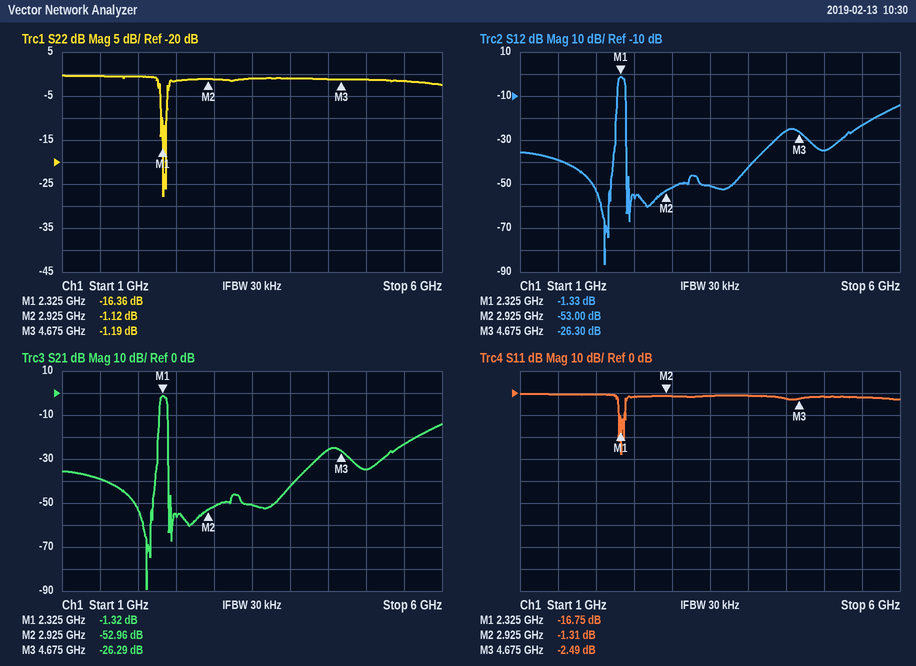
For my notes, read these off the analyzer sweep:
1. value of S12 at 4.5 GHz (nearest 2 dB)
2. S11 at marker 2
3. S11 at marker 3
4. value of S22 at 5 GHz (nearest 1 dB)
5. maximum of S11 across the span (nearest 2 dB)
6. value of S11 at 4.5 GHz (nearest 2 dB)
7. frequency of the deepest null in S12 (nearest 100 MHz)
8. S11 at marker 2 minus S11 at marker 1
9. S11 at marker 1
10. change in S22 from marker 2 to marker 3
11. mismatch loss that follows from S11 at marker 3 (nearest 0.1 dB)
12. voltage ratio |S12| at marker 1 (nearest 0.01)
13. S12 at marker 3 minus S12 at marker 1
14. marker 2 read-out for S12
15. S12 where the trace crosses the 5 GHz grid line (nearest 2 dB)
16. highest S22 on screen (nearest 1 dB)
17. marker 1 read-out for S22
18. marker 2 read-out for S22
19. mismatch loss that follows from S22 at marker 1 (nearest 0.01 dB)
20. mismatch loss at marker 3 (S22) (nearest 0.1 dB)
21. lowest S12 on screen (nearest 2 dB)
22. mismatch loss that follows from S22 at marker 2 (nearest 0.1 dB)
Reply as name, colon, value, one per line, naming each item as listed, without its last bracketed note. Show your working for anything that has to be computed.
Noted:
value of S12 at 4.5 GHz: -26 dB
S11 at marker 2: -1.31 dB
S11 at marker 3: -2.49 dB
value of S22 at 5 GHz: -1 dB
maximum of S11 across the span: 0 dB
value of S11 at 4.5 GHz: -2 dB
frequency of the deepest null in S12: 2.1 GHz
S11 at marker 2 minus S11 at marker 1: -1.31 − (-16.75) = 15.44 dB
S11 at marker 1: -16.75 dB
change in S22 from marker 2 to marker 3: -1.19 − (-1.12) = -0.07 dB
mismatch loss that follows from S11 at marker 3: −10 log10(1 − 10^(-2.49/10)) ≈ 3.6 dB
voltage ratio |S12| at marker 1: 10^(-1.33/20) ≈ 0.86
S12 at marker 3 minus S12 at marker 1: -26.3 − (-1.33) = -24.97 dB
marker 2 read-out for S12: -53.00 dB
S12 where the trace crosses the 5 GHz grid line: -34 dB
highest S22 on screen: 0 dB
marker 1 read-out for S22: -16.36 dB
marker 2 read-out for S22: -1.12 dB
mismatch loss that follows from S22 at marker 1: −10 log10(1 − 10^(-16.36/10)) ≈ 0.10 dB
mismatch loss at marker 3 (S22): −10 log10(1 − 10^(-1.19/10)) ≈ 6.2 dB
lowest S12 on screen: -86 dB
mismatch loss that follows from S22 at marker 2: −10 log10(1 − 10^(-1.12/10)) ≈ 6.4 dB
